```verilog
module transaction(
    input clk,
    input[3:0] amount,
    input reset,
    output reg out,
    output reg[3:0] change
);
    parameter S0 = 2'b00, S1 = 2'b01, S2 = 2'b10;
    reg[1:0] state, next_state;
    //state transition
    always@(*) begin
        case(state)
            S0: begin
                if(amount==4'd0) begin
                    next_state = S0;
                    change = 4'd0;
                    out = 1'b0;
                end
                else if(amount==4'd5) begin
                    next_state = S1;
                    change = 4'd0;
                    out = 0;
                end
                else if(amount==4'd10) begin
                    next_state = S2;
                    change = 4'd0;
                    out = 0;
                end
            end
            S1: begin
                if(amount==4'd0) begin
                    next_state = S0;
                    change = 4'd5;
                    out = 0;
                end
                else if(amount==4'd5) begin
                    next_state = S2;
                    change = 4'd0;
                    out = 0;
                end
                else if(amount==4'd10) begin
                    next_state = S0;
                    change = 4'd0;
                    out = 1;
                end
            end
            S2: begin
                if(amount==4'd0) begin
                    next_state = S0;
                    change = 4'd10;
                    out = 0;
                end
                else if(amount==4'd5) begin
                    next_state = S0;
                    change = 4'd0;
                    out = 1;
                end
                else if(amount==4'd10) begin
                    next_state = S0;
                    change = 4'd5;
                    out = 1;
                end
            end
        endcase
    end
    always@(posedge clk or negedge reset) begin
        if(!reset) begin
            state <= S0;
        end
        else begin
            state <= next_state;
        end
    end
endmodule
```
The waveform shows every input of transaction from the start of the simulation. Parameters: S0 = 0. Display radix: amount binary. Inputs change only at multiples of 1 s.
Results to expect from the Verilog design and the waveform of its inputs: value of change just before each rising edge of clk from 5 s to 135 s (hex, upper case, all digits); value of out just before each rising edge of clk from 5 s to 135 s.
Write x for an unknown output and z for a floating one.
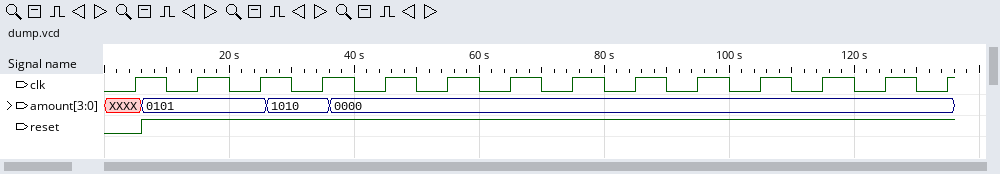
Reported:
x, 0, 0, 5, 0, 0, 0, 0, 0, 0, 0, 0, 0, 0
x 0 0 1 0 0 0 0 0 0 0 0 0 0
